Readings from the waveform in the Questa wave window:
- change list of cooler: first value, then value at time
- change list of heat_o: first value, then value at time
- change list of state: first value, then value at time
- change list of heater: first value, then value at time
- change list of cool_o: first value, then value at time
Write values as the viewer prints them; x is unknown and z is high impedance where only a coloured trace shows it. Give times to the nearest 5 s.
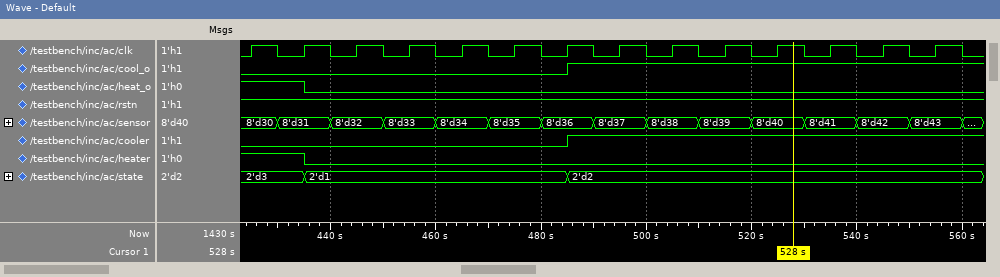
0, 1 at 485 s
1, 0 at 435 s
2'd3, 2'd1 at 435 s, 2'd2 at 485 s
1, 0 at 435 s
0, 1 at 485 s
